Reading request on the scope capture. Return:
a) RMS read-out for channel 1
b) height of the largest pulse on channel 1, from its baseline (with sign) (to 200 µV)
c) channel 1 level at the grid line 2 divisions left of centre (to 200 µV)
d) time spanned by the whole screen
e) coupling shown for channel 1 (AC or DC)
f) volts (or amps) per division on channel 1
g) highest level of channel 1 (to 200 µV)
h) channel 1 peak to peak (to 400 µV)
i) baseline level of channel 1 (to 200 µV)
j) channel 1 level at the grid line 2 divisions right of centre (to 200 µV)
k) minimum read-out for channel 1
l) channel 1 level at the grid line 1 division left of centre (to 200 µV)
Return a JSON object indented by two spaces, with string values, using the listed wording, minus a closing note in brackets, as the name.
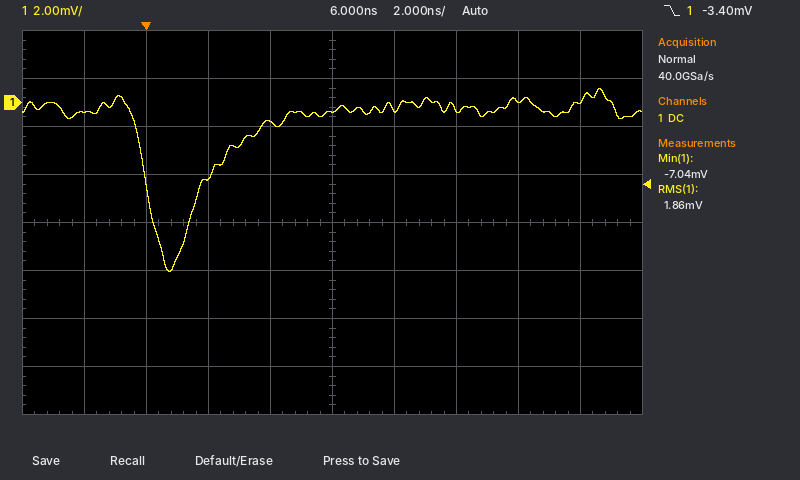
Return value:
{
  "RMS read-out for channel 1": "1.86 mV",
  "height of the largest pulse on channel 1, from its baseline (with sign)": "-6.6 mV",
  "channel 1 level at the grid line 2 divisions left of centre": "-3.2 mV",
  "time spanned by the whole screen": "20 ns",
  "coupling shown for channel 1": "DC",
  "volts (or amps) per division on channel 1": "2 mV",
  "highest level of channel 1": "600 µV",
  "channel 1 peak to peak": "7.6 mV",
  "baseline level of channel 1": "-400 µV",
  "channel 1 level at the grid line 2 divisions right of centre": "-200 µV",
  "minimum read-out for channel 1": "-7.04 mV",
  "channel 1 level at the grid line 1 division left of centre": "-800 µV"
}
